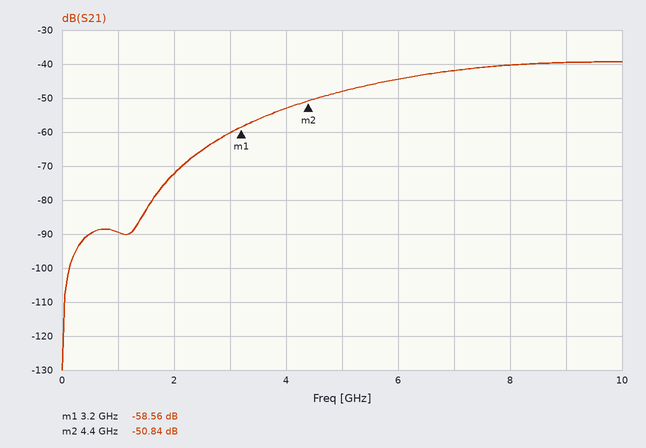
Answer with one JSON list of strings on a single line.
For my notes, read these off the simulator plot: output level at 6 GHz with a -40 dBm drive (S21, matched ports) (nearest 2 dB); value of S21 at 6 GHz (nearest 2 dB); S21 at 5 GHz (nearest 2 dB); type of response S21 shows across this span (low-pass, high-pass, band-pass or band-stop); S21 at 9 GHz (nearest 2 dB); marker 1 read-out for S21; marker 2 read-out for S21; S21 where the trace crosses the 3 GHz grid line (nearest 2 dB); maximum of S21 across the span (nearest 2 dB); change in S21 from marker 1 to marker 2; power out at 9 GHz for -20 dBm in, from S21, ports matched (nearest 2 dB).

["-84 dBm", "-44 dB", "-48 dB", "high-pass", "-40 dB", "-58.56 dB", "-50.84 dB", "-60 dB", "-40 dB", "7.72 dB", "-60 dBm"]
